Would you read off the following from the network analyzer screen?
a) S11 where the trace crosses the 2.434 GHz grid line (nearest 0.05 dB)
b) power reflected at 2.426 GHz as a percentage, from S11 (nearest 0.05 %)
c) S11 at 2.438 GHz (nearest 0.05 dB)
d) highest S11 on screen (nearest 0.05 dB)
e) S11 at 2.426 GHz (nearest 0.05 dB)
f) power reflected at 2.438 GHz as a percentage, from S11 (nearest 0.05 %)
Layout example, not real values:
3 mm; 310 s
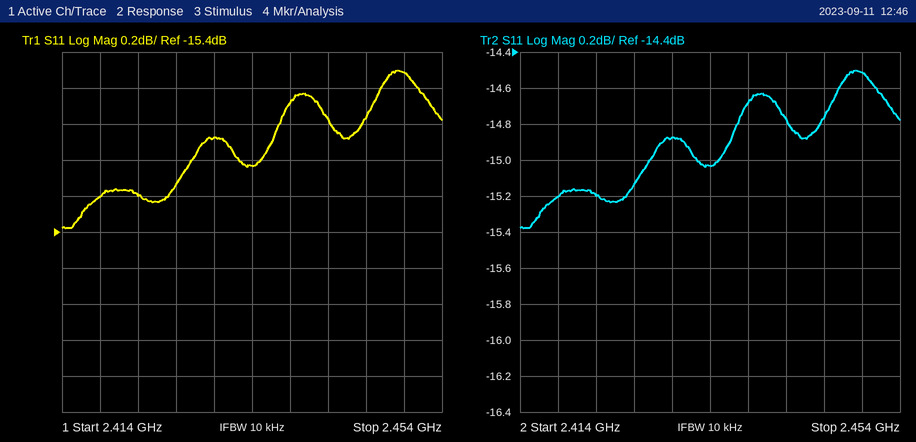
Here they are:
-15.05 dB; 3.05 %; -14.70 dB; -14.50 dB; -15.15 dB; 3.40 %
